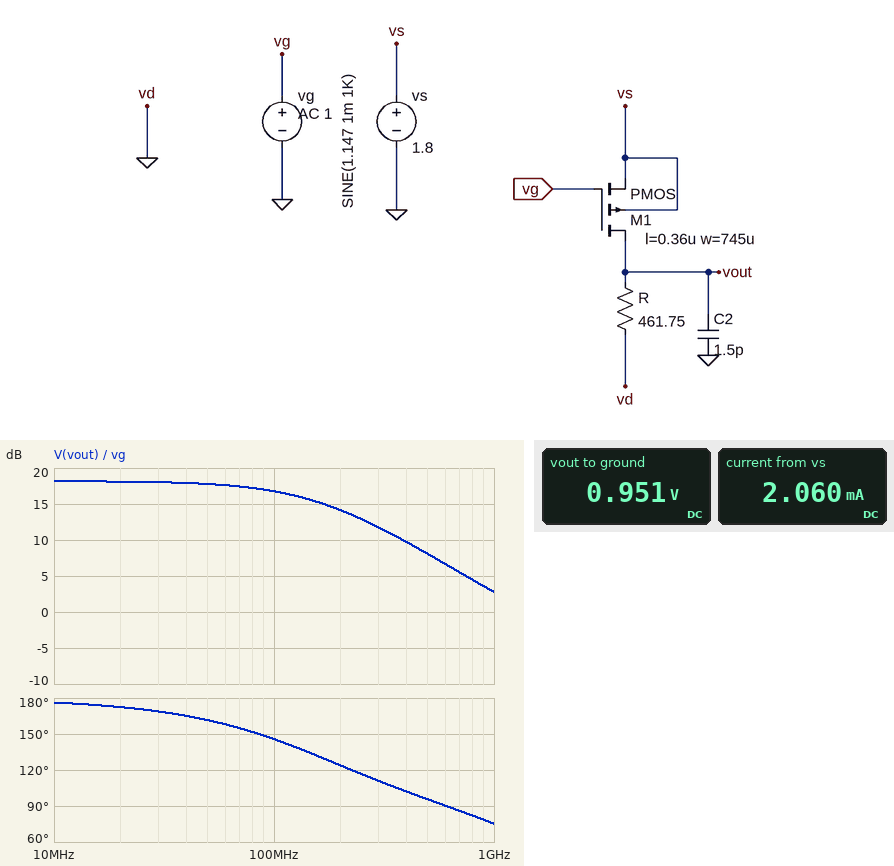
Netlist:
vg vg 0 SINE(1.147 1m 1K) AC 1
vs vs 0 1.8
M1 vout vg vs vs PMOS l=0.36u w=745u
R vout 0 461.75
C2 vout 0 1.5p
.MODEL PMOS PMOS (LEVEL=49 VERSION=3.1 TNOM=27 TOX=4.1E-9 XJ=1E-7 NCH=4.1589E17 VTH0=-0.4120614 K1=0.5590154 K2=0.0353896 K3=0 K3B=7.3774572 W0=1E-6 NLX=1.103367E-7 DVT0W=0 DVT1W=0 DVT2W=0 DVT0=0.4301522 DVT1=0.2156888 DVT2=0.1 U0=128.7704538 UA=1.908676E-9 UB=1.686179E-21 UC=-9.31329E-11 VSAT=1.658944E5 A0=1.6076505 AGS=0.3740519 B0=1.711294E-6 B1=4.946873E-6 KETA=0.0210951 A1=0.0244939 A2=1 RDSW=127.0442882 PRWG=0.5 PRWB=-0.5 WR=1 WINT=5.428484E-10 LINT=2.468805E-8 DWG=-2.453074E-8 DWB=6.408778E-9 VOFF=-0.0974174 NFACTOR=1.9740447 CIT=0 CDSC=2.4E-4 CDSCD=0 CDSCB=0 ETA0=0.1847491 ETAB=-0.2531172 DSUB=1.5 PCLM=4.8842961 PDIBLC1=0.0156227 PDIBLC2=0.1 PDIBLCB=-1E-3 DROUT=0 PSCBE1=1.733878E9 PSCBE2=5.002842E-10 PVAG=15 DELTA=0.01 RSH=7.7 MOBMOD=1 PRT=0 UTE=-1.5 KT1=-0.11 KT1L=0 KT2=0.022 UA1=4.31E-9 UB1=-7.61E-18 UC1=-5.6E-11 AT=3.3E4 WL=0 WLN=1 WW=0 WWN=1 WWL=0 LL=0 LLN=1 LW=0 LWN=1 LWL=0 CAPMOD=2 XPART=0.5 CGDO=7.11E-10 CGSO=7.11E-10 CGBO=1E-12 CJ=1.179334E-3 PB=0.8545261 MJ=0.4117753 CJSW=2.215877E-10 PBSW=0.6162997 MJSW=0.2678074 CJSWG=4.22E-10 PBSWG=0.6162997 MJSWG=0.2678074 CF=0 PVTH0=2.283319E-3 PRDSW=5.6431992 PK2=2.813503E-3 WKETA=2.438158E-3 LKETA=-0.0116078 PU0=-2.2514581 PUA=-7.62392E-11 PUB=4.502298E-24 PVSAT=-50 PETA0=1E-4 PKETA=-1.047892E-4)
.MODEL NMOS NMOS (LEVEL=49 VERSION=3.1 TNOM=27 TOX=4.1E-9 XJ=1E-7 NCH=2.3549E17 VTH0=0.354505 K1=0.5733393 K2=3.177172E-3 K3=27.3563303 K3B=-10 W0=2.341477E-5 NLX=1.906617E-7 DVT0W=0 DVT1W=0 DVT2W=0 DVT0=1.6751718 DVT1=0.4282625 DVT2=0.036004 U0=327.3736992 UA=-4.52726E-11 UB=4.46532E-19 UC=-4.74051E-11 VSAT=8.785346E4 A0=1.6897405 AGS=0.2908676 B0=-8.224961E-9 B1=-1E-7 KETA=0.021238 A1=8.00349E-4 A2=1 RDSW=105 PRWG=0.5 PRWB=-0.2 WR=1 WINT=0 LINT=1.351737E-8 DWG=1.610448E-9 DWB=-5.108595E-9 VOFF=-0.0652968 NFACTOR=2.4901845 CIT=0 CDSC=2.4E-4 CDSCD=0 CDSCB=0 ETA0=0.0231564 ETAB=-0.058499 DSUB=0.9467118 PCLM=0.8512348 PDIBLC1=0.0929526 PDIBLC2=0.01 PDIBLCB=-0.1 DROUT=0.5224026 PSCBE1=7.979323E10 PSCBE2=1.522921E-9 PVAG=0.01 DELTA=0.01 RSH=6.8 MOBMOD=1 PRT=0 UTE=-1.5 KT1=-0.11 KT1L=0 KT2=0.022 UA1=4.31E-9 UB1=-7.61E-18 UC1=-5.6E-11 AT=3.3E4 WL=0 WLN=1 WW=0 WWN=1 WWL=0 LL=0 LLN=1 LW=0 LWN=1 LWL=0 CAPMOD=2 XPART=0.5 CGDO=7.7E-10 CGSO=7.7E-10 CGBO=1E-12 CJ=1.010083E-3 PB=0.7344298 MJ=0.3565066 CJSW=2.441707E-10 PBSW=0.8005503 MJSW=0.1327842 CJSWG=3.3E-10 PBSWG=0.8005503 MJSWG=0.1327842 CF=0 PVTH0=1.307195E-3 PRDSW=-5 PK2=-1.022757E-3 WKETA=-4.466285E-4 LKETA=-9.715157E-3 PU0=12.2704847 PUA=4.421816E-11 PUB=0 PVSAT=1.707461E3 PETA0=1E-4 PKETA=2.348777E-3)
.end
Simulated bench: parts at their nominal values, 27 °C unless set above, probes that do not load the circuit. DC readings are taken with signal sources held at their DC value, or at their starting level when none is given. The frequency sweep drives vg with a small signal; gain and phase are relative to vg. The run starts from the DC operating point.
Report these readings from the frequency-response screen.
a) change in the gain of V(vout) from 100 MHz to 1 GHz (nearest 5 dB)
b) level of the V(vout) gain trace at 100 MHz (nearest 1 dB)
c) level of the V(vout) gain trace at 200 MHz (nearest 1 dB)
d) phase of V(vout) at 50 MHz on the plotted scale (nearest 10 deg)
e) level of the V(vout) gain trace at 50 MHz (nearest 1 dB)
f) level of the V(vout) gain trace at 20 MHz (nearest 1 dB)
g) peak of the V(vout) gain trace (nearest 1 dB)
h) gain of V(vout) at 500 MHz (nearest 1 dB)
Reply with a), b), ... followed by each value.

a) -15 dB
b) 17 dB
c) 14 dB
d) 160 deg
e) 18 dB
f) 18 dB
g) 18 dB
h) 8 dB
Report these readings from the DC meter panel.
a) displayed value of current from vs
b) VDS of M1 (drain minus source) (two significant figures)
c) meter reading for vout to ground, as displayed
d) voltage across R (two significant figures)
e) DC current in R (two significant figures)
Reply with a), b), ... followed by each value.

a) 2.060 mA
b) -850 mV
c) 0.951 V
d) 950 mV
e) 2.1 mA
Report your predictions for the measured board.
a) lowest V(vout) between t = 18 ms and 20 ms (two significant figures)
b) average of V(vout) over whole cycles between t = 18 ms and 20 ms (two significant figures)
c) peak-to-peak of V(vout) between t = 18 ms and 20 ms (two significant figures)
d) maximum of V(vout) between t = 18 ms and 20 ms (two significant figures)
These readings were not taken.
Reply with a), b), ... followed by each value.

a) 940 mV
b) 950 mV
c) 16 mV
d) 960 mV
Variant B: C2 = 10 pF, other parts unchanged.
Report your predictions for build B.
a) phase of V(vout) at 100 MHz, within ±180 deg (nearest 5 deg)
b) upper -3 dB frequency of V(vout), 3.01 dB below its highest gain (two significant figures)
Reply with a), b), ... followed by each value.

a) 105 deg
b) 34 MHz
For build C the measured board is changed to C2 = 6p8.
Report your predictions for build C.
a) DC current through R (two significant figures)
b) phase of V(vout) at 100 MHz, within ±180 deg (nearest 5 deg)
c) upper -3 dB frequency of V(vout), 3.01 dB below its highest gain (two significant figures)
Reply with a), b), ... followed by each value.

a) 2.1 mA
b) 115 deg
c) 49 MHz
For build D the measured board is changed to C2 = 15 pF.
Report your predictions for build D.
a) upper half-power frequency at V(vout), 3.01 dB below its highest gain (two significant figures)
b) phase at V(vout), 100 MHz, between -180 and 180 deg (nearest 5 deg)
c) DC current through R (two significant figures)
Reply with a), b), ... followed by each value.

a) 23 MHz
b) 100 deg
c) 2.1 mA
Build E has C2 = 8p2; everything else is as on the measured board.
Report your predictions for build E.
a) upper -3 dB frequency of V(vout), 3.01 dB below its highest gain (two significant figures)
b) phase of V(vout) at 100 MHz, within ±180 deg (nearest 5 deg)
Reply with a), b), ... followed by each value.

a) 41 MHz
b) 110 deg
